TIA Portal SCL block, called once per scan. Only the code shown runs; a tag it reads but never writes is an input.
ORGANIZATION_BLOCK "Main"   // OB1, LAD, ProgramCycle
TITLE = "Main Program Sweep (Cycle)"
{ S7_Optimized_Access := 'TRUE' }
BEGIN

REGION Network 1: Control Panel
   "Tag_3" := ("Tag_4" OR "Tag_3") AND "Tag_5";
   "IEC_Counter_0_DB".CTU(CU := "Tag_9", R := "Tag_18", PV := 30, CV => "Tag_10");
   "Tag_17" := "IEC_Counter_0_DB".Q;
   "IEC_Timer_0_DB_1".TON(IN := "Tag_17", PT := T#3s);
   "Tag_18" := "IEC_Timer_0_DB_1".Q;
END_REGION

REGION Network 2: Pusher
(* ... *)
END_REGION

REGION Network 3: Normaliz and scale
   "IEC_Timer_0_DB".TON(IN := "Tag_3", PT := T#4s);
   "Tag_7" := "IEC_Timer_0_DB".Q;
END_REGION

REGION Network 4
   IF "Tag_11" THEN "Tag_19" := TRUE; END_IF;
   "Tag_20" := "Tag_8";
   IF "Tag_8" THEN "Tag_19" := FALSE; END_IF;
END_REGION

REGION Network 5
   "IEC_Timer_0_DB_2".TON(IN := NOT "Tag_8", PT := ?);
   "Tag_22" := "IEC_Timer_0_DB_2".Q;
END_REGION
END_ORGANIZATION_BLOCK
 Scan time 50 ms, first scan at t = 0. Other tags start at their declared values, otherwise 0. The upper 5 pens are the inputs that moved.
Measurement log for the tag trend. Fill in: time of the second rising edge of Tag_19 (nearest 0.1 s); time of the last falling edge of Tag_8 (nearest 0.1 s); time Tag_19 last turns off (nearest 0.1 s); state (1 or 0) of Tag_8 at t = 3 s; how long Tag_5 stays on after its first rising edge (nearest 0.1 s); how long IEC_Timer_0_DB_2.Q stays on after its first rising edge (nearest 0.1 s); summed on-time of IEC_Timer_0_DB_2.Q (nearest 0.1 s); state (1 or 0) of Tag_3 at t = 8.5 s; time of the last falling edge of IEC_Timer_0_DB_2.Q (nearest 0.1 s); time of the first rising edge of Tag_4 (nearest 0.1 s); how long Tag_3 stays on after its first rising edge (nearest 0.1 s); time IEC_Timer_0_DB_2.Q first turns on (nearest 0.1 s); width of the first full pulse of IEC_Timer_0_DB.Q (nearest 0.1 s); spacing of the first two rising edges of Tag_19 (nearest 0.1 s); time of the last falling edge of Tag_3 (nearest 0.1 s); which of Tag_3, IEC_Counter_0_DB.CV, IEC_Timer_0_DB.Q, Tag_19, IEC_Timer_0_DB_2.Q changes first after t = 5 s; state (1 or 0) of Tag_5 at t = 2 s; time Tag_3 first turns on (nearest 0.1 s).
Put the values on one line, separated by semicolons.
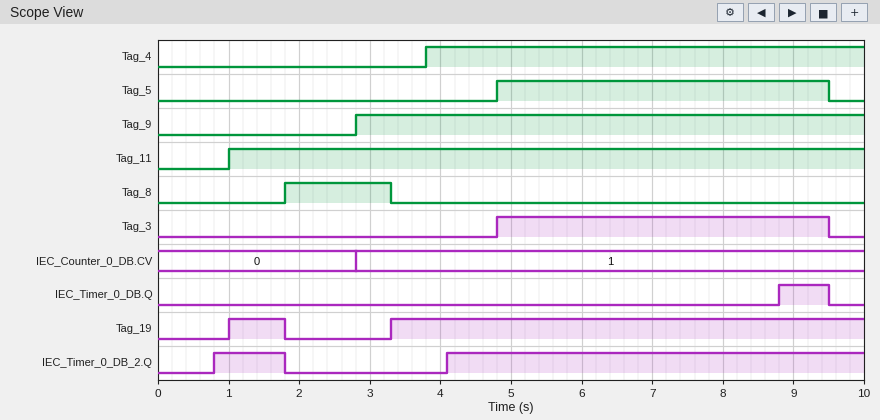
3.3 s; 3.3 s; 1.8 s; 1; 4.7 s; 1.0 s; 6.9 s; 1; 1.8 s; 3.8 s; 4.7 s; 0.8 s; 0.7 s; 2.3 s; 9.5 s; IEC_Timer_0_DB.Q; 0; 4.8 s
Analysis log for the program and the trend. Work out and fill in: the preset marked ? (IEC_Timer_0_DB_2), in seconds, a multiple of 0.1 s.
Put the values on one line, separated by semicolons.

0.8 s
